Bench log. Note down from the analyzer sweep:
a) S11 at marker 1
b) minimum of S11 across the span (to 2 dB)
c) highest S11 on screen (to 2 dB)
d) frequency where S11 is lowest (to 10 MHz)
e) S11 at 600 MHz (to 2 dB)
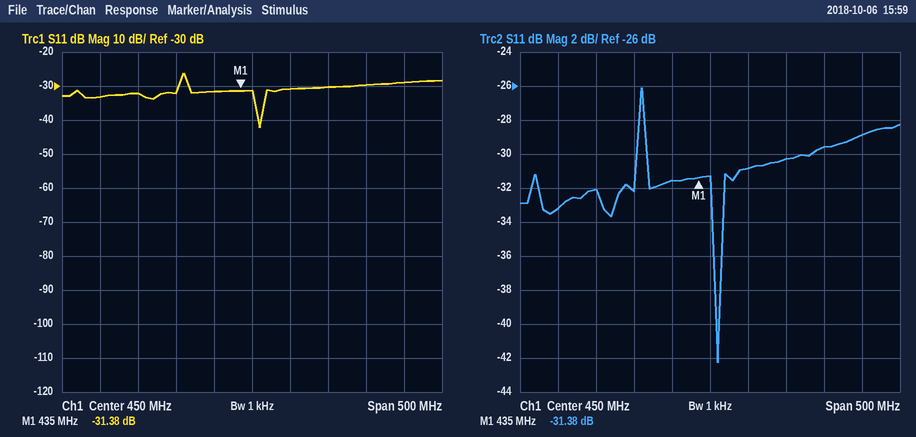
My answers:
-31.38 dB
-42 dB
-26 dB
460 MHz
-30 dB
